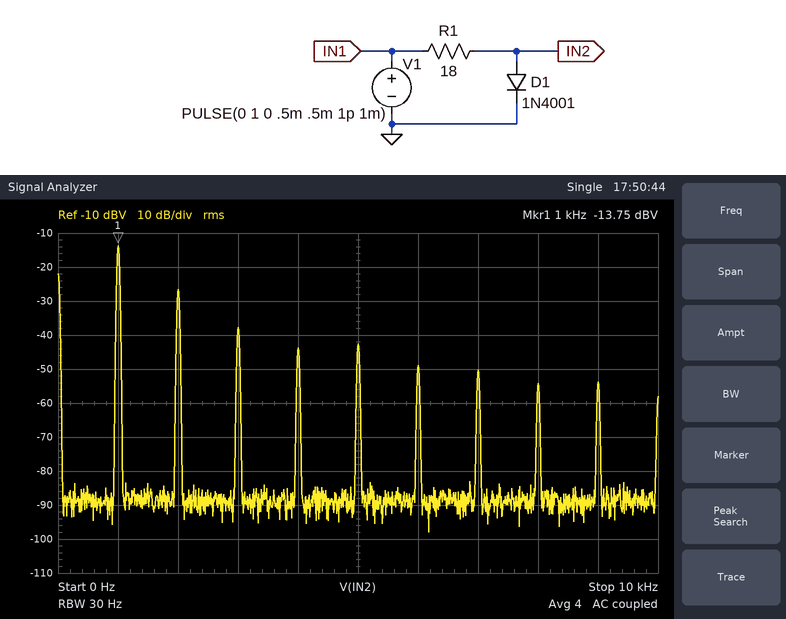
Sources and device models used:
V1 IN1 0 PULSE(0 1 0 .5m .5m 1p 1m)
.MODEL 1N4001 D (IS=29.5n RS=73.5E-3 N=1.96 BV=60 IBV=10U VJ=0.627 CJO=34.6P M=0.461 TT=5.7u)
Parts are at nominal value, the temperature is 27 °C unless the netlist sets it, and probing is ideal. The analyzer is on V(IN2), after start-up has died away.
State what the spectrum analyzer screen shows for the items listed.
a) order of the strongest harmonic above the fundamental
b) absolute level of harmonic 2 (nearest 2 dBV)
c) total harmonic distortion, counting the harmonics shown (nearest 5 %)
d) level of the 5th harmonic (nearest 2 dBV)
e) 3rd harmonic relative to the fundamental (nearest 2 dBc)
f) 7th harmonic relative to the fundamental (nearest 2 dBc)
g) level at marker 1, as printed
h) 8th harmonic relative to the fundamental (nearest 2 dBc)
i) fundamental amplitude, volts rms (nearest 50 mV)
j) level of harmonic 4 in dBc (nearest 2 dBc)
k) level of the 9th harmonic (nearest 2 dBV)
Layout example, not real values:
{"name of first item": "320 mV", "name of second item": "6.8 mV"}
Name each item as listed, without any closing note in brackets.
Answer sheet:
{"order of the strongest harmonic above the fundamental": "2", "absolute level of harmonic 2": "-26 dBV", "total harmonic distortion, counting the harmonics shown": "25 %", "level of the 5th harmonic": "-42 dBV", "3rd harmonic relative to the fundamental": "-24 dBc", "7th harmonic relative to the fundamental": "-36 dBc", "level at marker 1, as printed": "-13.75 dBV", "8th harmonic relative to the fundamental": "-40 dBc", "fundamental amplitude, volts rms": "200 mV", "level of harmonic 4 in dBc": "-30 dBc", "level of the 9th harmonic": "-54 dBV"}
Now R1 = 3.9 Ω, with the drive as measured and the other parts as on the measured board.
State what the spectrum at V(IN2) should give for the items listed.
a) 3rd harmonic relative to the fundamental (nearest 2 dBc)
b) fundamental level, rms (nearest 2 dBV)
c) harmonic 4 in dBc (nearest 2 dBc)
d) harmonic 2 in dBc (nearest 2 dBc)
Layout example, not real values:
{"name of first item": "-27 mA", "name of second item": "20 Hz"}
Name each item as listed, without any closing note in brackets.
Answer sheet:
{"3rd harmonic relative to the fundamental": "-26 dBc", "fundamental level, rms": "-12 dBV", "harmonic 4 in dBc": "-28 dBc", "harmonic 2 in dBc": "-16 dBc"}
